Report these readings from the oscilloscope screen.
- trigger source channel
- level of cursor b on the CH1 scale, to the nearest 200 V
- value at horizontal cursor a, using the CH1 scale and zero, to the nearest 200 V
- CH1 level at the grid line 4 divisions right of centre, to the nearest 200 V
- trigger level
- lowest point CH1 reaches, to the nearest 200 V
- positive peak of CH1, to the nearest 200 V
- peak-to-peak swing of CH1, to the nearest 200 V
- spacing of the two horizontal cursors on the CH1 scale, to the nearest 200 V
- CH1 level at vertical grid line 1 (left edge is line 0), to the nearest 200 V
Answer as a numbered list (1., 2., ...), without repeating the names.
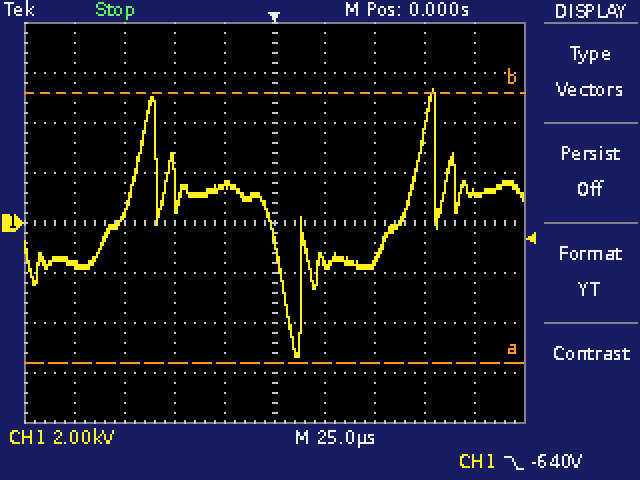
1. CH1
2. 5.2 kV
3. -5.6 kV
4. 1.2 kV
5. -640 V
6. -5.4 kV
7. 5.4 kV
8. 10.8 kV
9. 10.8 kV
10. -1.6 kV
